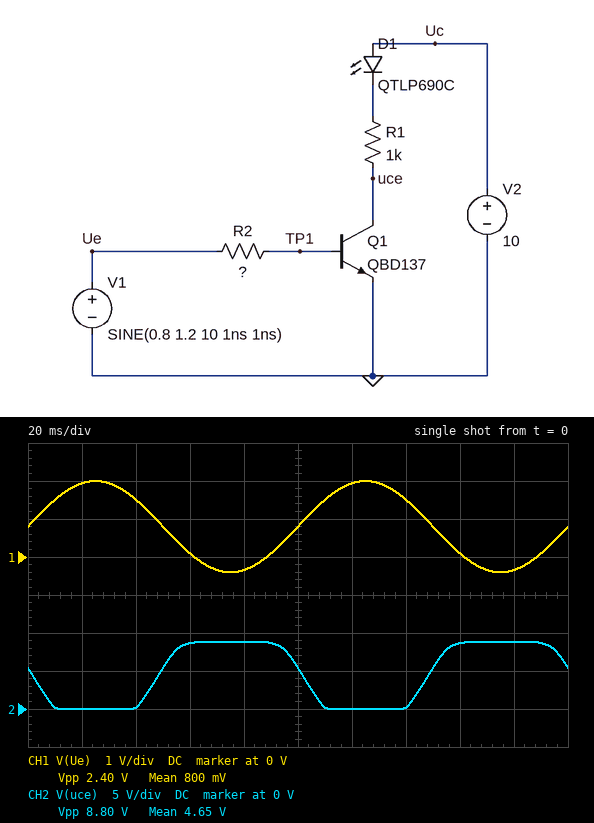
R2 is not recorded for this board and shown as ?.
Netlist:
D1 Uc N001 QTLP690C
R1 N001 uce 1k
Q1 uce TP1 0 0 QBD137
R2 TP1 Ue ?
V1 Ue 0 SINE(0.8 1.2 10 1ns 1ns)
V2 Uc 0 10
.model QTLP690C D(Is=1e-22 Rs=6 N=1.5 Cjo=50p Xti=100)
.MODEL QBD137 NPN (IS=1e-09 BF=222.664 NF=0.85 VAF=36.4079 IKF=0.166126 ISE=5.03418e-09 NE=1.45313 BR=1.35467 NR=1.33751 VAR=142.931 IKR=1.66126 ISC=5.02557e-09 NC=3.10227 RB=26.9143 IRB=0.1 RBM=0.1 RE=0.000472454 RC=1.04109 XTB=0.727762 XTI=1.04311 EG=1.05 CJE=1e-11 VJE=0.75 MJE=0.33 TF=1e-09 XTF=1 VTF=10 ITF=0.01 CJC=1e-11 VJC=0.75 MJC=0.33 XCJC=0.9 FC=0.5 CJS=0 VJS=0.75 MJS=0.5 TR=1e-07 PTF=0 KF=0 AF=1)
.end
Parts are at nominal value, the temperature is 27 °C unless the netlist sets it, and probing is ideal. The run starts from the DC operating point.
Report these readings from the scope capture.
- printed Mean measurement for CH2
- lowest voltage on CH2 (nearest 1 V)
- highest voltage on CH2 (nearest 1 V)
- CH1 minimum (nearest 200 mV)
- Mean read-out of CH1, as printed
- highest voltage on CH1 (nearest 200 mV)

4.65 V
0 V
9 V
-400 mV
800 mV
2.0 V
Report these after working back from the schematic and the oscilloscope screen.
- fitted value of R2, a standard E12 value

12 kΩ
